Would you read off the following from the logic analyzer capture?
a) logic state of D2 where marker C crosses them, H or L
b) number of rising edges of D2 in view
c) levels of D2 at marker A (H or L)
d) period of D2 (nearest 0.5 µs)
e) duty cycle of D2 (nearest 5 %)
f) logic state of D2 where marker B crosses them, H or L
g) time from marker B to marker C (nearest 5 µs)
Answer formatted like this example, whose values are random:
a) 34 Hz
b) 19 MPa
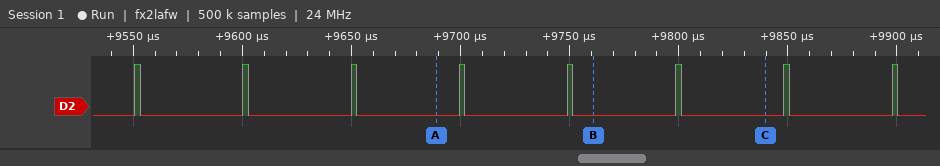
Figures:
a) D2=L
b) 8
c) D2=L
d) 49.5 µs
e) 5 %
f) D2=L
g) 80 µs
